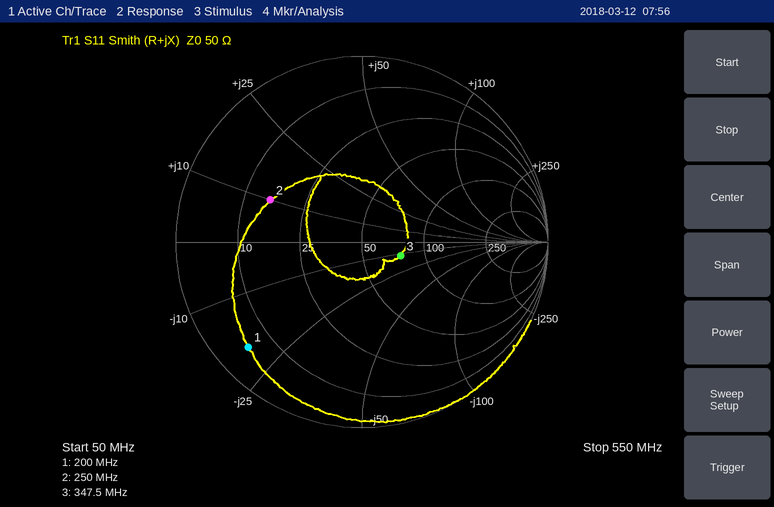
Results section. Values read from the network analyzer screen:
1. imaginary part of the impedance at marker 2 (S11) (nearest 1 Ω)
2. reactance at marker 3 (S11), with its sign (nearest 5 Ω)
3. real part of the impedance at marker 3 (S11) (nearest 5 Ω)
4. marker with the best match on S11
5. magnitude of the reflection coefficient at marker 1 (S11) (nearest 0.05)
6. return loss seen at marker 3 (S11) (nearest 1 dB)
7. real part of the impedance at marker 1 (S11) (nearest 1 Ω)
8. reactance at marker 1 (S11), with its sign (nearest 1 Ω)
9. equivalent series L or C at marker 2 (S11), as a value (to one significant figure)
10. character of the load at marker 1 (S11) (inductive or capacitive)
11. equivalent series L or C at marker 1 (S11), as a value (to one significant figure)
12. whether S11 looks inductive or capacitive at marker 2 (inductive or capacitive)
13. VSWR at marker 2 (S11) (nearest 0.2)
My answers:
+10 Ω
-10 Ω
75 Ω
marker 3
0.85
13 dB
5 Ω
-19 Ω
6 nH
capacitive
40 pF
inductive
3.4
